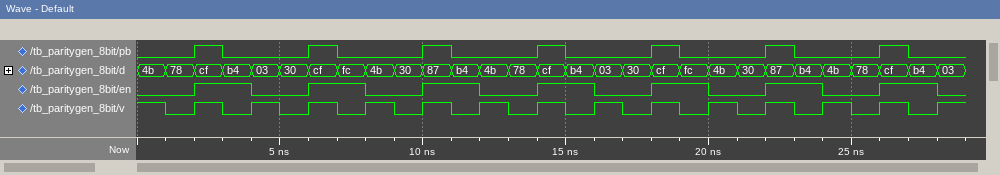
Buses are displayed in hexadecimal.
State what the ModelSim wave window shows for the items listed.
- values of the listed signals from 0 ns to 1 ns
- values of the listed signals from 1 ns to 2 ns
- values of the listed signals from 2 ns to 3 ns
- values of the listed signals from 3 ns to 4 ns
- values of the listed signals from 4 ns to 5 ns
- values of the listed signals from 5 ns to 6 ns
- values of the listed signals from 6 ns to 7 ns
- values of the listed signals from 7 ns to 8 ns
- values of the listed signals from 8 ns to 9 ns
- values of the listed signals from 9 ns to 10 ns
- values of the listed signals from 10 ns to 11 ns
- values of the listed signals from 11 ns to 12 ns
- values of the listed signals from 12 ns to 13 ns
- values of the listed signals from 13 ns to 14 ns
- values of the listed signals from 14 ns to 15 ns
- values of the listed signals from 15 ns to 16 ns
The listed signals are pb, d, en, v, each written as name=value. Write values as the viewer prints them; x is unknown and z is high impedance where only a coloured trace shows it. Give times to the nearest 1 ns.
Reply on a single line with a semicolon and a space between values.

pb=0, d=4b, en=0, v=1; pb=0, d=78, en=0, v=0; pb=1, d=cf, en=1, v=1; pb=0, d=b4, en=1, v=0; pb=0, d=03, en=0, v=1; pb=0, d=30, en=0, v=0; pb=1, d=cf, en=1, v=1; pb=0, d=fc, en=1, v=0; pb=0, d=4b, en=0, v=1; pb=0, d=30, en=0, v=0; pb=1, d=87, en=1, v=1; pb=0, d=b4, en=1, v=0; pb=0, d=4b, en=0, v=1; pb=0, d=78, en=0, v=0; pb=1, d=cf, en=1, v=1; pb=0, d=b4, en=1, v=0
